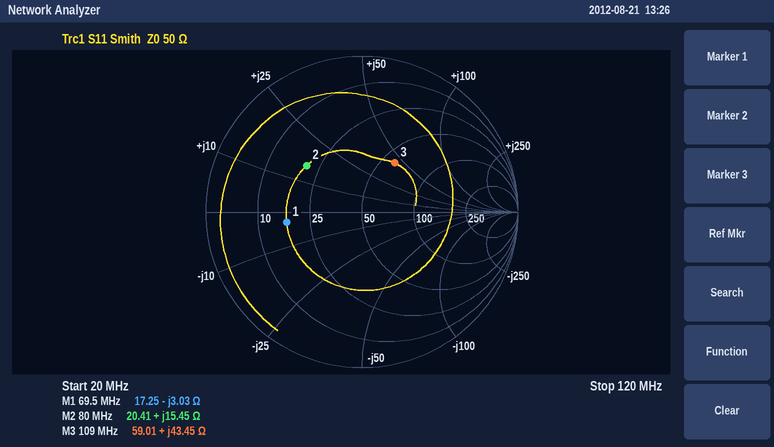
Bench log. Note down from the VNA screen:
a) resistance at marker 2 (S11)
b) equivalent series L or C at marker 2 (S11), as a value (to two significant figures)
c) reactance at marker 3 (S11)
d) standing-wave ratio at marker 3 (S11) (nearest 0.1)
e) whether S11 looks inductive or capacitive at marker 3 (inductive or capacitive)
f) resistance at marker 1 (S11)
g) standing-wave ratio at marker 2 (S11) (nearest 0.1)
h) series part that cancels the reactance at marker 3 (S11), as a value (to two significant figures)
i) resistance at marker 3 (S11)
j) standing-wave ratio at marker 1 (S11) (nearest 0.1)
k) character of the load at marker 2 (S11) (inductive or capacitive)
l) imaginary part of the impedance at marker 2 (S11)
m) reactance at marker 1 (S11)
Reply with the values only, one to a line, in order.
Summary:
20.41 Ω
31 nH
+43.45 Ω
2.2
inductive
17.25 Ω
2.7
34 pF
59.01 Ω
2.9
inductive
+15.45 Ω
-3.03 Ω
